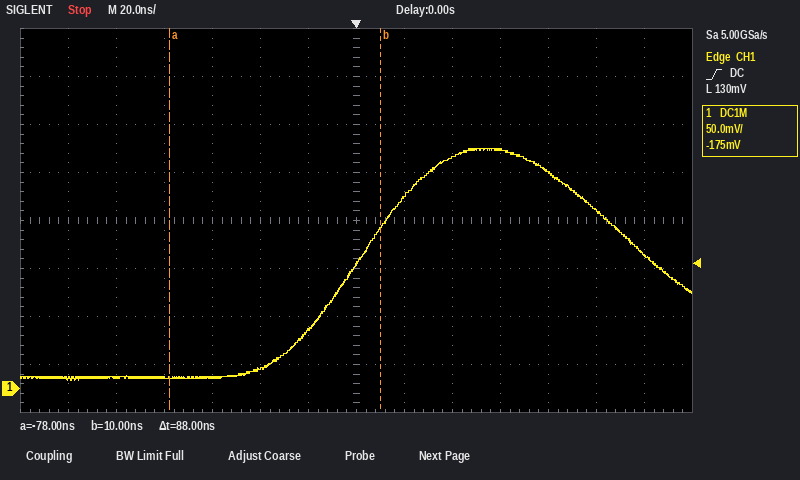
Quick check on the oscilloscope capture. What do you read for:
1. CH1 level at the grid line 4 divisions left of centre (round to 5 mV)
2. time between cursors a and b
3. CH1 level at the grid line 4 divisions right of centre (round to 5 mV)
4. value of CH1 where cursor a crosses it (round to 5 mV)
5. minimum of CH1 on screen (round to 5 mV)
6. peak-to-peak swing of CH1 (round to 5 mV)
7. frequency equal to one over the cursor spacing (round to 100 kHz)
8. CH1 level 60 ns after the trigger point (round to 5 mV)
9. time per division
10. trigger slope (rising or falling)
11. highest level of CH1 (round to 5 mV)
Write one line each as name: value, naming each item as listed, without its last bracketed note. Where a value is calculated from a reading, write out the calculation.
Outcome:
CH1 level at the grid line 4 divisions left of centre: 10 mV
time between cursors a and b: 88 ns
CH1 level at the grid line 4 divisions right of centre: 225 mV
value of CH1 where cursor a crosses it: 10 mV
minimum of CH1 on screen: 10 mV
peak-to-peak swing of CH1: 250 mV − (10 mV) = 240 mV
frequency equal to one over the cursor spacing: 1 / 88 ns ≈ 11.4 MHz
CH1 level 60 ns after the trigger point: 250 mV
time per division: 20 ns
trigger slope: rising
highest level of CH1: 250 mV
